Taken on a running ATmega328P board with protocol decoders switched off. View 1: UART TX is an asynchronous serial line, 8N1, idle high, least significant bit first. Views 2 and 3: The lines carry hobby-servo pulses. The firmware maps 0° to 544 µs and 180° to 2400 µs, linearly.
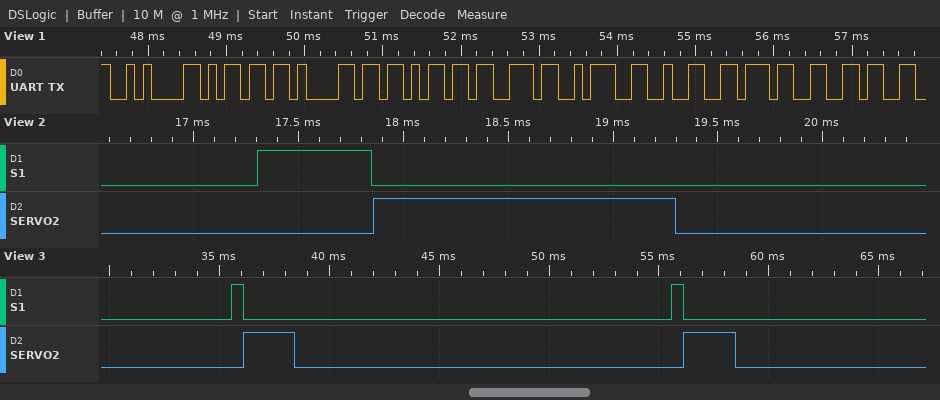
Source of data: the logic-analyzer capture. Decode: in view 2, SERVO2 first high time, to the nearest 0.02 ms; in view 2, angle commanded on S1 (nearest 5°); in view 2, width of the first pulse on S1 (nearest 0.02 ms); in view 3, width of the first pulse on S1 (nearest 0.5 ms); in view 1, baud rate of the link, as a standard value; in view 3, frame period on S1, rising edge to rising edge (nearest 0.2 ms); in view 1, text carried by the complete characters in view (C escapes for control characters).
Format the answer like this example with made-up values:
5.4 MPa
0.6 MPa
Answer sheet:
1.44 ms
0°
0.54 ms
0.5 ms
9600 baud
20.0 ms
"\nmaks:276"
